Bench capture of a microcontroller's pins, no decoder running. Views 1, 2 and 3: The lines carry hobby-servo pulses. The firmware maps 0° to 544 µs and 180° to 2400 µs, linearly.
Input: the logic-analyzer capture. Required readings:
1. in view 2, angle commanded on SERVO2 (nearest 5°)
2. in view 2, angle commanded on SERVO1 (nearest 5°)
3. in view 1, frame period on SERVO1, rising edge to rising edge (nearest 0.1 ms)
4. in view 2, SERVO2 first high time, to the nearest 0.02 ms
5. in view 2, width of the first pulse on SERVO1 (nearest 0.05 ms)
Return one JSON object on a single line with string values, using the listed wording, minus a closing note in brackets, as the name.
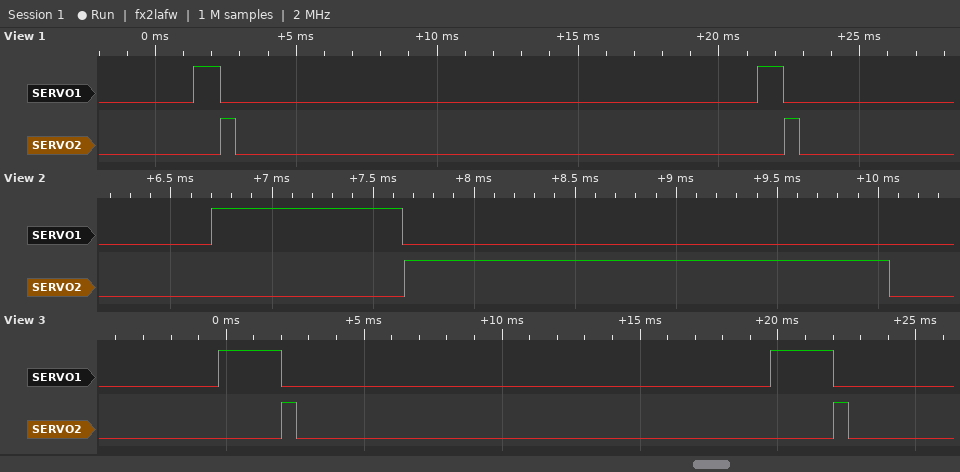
{"in view 2, angle commanded on SERVO2": "180°", "in view 2, angle commanded on SERVO1": "40°", "in view 1, frame period on SERVO1, rising edge to rising edge": "20.0 ms", "in view 2, SERVO2 first high time, to the nearest 0.02 ms": "2.40 ms", "in view 2, width of the first pulse on SERVO1": "0.95 ms"}
